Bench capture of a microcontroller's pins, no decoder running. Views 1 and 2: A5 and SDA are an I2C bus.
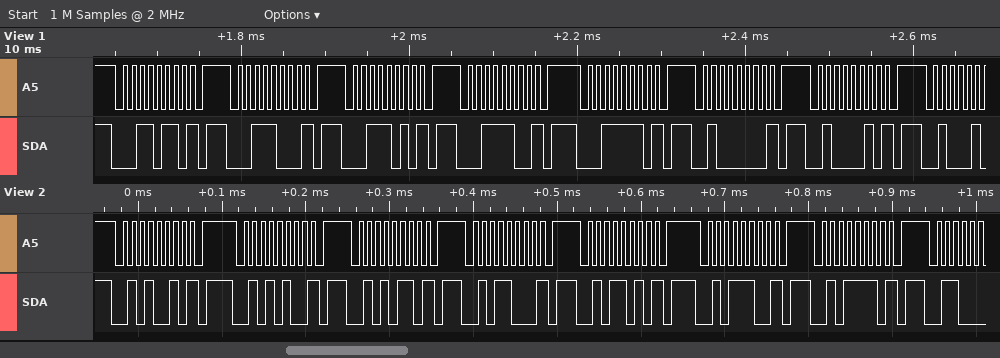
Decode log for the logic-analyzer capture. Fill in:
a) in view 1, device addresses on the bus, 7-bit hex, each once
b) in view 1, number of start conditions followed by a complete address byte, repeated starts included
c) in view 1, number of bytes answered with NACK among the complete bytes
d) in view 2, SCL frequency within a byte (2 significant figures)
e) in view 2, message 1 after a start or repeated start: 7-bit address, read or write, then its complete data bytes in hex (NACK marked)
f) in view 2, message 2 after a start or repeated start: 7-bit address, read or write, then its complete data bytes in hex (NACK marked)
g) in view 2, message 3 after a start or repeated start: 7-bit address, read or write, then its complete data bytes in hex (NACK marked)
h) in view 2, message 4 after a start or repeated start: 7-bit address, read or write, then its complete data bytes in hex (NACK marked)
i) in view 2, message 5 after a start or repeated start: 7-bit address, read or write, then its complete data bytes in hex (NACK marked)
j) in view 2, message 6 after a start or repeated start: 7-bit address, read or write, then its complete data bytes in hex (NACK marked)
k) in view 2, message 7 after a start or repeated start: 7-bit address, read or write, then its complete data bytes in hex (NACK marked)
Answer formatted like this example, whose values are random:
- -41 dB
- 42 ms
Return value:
- 0x1B 0x1C 0x1D 0x1E 0x1F 0x20 0x21
- 7
- 7
- 100 kHz
- 0x29 write NACK
- 0x2A write NACK
- 0x2B write NACK
- 0x2C write NACK
- 0x2D write NACK
- 0x2E write NACK
- 0x2F write NACK
